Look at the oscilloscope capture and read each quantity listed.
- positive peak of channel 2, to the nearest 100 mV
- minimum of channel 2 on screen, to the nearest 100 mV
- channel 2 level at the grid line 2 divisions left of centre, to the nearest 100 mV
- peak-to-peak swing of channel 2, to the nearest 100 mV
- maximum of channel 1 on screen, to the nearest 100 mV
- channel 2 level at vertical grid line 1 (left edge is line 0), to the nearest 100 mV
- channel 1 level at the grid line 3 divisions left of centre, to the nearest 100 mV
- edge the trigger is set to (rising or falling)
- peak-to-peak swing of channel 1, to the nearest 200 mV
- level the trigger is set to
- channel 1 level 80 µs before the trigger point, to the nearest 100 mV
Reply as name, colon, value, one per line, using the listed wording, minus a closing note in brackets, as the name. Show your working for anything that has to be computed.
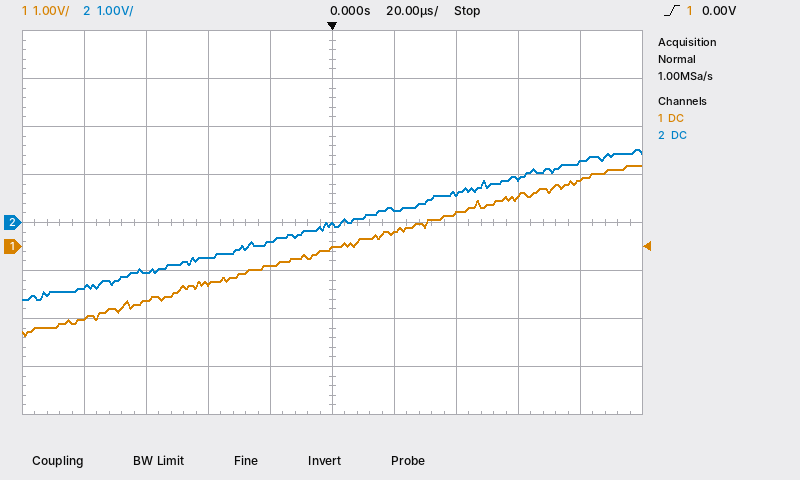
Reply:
positive peak of channel 2, to the nearest 100 mV: 1.5 V
minimum of channel 2 on screen, to the nearest 100 mV: -1.6 V
channel 2 level at the grid line 2 divisions left of centre, to the nearest 100 mV: -700 mV
peak-to-peak swing of channel 2, to the nearest 100 mV: 1.5 V − (-1.6 V) = 3.1 V
maximum of channel 1 on screen, to the nearest 100 mV: 1.7 V
channel 2 level at vertical grid line 1 (left edge is line 0), to the nearest 100 mV: -1.3 V
channel 1 level at the grid line 3 divisions left of centre, to the nearest 100 mV: -1.1 V
edge the trigger is set to: rising
peak-to-peak swing of channel 1, to the nearest 200 mV: 3.6 V
level the trigger is set to: 0.00 V
channel 1 level 80 µs before the trigger point, to the nearest 100 mV: -1.5 V
